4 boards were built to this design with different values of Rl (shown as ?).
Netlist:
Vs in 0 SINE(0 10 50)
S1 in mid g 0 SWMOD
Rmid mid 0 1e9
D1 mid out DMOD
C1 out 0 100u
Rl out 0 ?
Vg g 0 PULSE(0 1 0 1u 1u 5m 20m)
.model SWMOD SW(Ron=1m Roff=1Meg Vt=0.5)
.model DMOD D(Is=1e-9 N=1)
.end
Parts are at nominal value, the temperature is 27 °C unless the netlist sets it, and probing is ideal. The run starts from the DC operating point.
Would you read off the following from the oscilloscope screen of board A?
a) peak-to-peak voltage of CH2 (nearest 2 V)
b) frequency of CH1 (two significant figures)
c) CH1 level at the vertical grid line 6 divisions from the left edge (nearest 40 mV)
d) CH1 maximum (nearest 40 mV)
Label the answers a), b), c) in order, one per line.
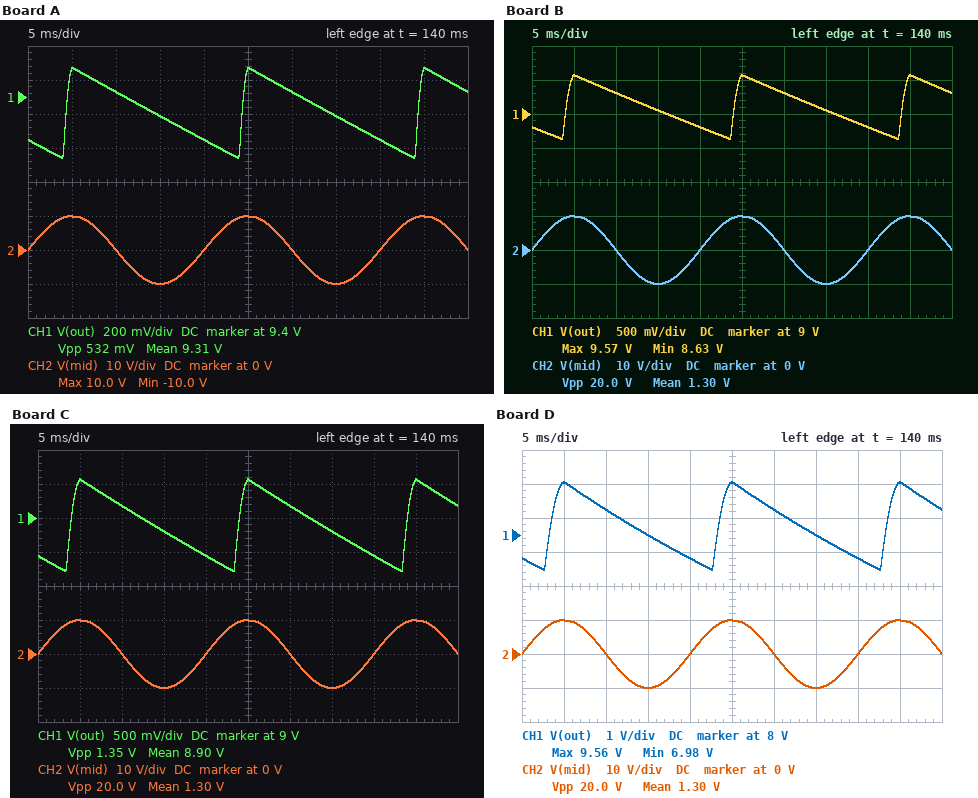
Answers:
a) 20 V
b) 50 Hz
c) 9.44 V
d) 9.56 V
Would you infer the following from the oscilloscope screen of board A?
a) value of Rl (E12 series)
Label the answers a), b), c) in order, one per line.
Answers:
a) 3.3 kΩ
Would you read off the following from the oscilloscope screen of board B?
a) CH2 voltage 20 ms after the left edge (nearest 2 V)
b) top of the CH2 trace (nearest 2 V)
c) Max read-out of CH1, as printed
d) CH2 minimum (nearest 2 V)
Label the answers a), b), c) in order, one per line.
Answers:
a) 0 V
b) 10 V
c) 9.57 V
d) -10 V
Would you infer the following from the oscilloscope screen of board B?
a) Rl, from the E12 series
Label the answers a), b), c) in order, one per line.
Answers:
a) 1.8 kΩ
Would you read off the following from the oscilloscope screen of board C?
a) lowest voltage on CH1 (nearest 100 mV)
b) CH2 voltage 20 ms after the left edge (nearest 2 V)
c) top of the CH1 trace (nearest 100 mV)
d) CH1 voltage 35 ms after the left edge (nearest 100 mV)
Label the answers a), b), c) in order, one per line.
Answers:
a) 8.2 V
b) 0 V
c) 9.6 V
d) 8.8 V
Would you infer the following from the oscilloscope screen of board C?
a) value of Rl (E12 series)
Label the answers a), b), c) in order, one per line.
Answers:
a) 1.2 kΩ
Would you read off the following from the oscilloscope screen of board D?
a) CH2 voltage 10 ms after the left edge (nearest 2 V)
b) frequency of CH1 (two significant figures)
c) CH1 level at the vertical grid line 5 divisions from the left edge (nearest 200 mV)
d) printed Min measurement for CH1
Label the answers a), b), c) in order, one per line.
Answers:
a) 0 V
b) 50 Hz
c) 9.6 V
d) 6.98 V
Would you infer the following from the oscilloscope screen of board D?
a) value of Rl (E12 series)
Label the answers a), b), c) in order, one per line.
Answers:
a) 560 Ω
